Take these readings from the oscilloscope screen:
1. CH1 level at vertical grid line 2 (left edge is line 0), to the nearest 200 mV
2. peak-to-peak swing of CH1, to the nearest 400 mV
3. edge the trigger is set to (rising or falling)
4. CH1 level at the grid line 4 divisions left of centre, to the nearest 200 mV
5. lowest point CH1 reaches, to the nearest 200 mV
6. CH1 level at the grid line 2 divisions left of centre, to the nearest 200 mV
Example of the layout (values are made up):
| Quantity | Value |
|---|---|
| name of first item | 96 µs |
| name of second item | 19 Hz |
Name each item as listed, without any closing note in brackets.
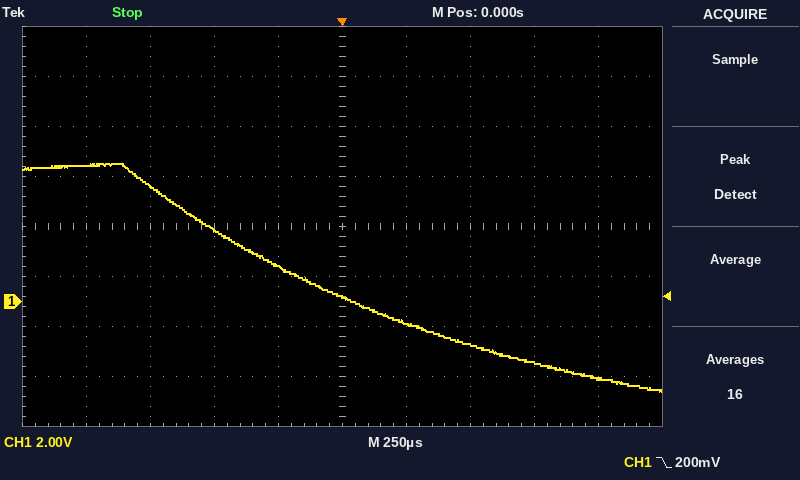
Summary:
| Quantity | Value |
|---|---|
| CH1 level at vertical grid line 2 (left edge is line 0), to the nearest 200 mV | 4.6 V |
| peak-to-peak swing of CH1, to the nearest 400 mV | 9.2 V |
| edge the trigger is set to | falling |
| CH1 level at the grid line 4 divisions left of centre, to the nearest 200 mV | 5.4 V |
| lowest point CH1 reaches, to the nearest 200 mV | -3.6 V |
| CH1 level at the grid line 2 divisions left of centre, to the nearest 200 mV | 2.8 V |
